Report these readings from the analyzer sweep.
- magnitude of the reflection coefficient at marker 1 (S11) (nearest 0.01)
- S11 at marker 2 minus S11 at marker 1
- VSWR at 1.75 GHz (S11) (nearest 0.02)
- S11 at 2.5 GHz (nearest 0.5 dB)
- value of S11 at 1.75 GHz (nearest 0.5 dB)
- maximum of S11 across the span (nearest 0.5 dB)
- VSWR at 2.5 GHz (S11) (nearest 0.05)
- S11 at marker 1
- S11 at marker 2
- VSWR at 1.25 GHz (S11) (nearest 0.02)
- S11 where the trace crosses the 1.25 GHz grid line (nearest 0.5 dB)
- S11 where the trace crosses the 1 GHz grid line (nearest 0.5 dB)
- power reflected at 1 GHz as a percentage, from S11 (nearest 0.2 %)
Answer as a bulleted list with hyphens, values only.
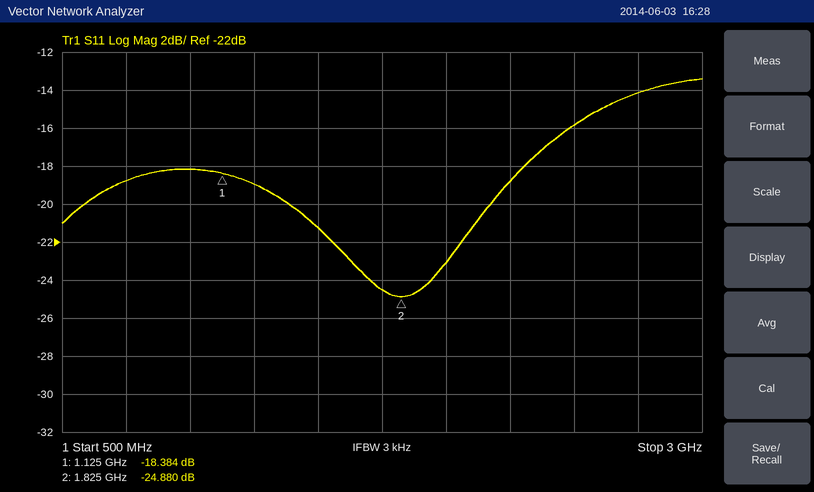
- 0.12
- -6.496 dB
- 1.12
- -16.0 dB
- -24.5 dB
- -13.5 dB
- 1.40
- -18.384 dB
- -24.880 dB
- 1.26
- -19.0 dB
- -18.0 dB
- 1.6 %
